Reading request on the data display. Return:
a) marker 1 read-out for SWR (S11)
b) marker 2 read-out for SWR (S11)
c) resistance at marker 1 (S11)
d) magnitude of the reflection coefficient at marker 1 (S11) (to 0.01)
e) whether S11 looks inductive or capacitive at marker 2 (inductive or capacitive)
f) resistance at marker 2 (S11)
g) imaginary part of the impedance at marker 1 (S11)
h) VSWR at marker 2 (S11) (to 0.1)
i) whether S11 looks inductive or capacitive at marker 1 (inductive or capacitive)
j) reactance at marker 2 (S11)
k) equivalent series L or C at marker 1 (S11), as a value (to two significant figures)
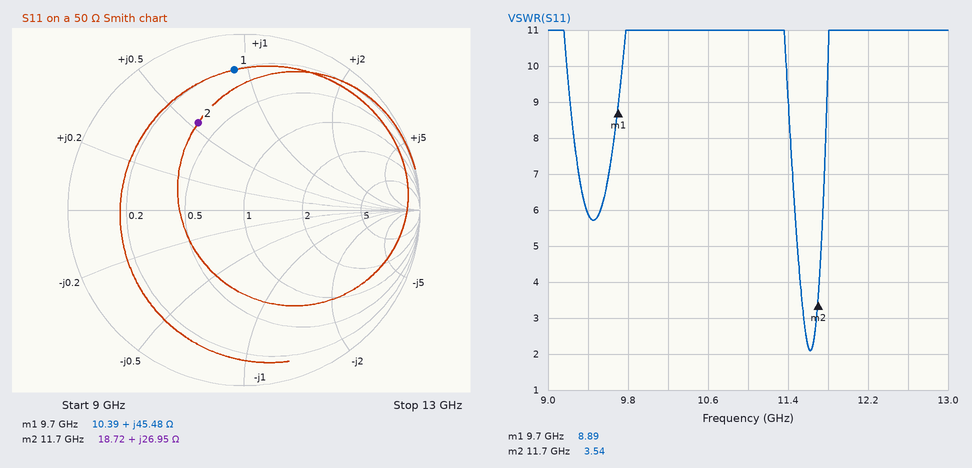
8.89
3.54
10.39 Ω
0.80
inductive
18.72 Ω
+45.48 Ω
3.5
inductive
+26.95 Ω
750 pH
